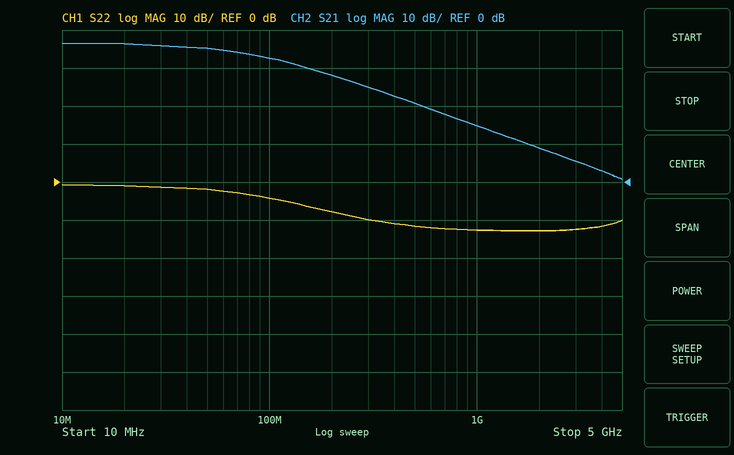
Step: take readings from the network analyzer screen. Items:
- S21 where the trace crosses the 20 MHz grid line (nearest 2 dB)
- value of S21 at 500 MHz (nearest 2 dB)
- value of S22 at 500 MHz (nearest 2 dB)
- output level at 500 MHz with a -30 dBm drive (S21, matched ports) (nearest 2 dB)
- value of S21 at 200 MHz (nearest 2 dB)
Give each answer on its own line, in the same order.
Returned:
36 dB
20 dB
-12 dB
-10 dBm
28 dB
